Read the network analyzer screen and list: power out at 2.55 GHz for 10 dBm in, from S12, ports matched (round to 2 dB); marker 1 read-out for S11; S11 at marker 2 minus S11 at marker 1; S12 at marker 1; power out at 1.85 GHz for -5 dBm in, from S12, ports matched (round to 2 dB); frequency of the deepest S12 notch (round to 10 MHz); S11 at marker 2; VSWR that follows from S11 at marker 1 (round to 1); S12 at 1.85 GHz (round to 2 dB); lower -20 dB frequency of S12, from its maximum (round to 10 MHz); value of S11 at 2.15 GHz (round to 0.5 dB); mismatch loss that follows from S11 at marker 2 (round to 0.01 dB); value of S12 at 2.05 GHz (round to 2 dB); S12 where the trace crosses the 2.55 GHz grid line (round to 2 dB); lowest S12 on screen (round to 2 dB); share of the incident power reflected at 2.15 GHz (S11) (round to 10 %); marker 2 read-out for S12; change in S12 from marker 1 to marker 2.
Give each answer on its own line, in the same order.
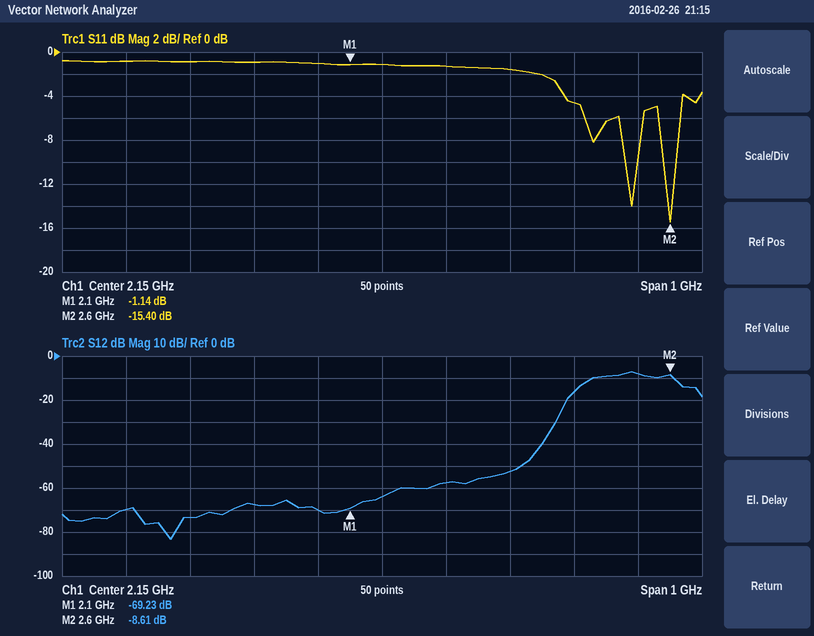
2 dBm
-1.14 dB
-14.26 dB
-69.23 dB
-78 dBm
1.82 GHz
-15.40 dB
15
-74 dB
2.43 GHz
-1.0 dB
0.13 dB
-70 dB
-8 dB
-84 dB
80 %
-8.61 dB
60.62 dB
